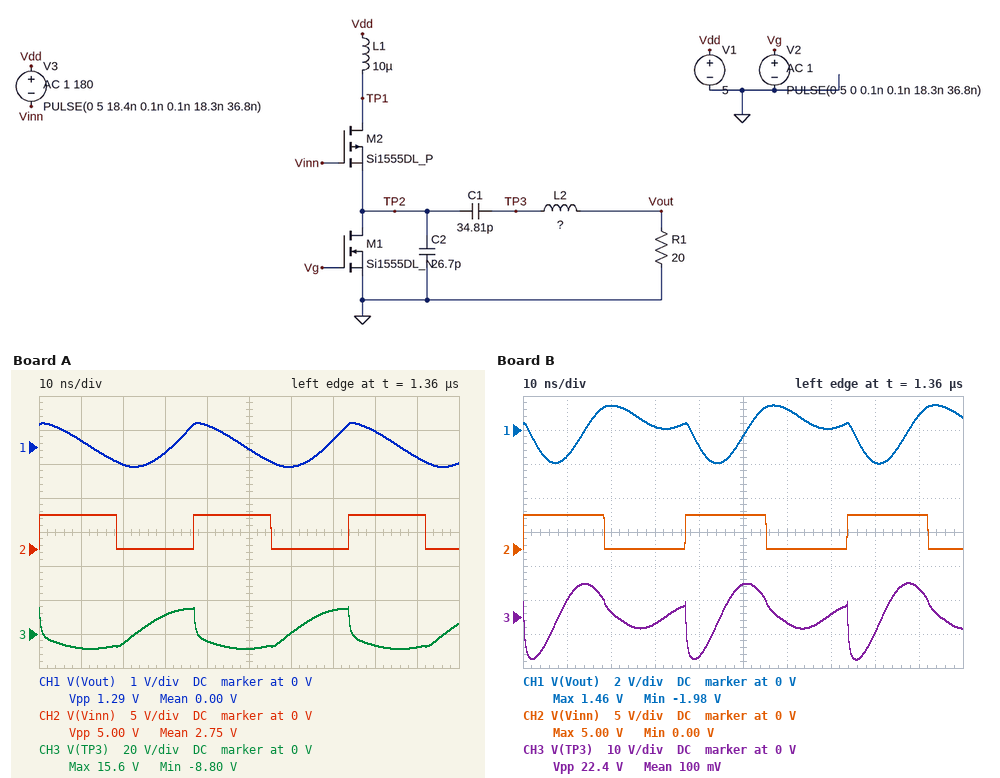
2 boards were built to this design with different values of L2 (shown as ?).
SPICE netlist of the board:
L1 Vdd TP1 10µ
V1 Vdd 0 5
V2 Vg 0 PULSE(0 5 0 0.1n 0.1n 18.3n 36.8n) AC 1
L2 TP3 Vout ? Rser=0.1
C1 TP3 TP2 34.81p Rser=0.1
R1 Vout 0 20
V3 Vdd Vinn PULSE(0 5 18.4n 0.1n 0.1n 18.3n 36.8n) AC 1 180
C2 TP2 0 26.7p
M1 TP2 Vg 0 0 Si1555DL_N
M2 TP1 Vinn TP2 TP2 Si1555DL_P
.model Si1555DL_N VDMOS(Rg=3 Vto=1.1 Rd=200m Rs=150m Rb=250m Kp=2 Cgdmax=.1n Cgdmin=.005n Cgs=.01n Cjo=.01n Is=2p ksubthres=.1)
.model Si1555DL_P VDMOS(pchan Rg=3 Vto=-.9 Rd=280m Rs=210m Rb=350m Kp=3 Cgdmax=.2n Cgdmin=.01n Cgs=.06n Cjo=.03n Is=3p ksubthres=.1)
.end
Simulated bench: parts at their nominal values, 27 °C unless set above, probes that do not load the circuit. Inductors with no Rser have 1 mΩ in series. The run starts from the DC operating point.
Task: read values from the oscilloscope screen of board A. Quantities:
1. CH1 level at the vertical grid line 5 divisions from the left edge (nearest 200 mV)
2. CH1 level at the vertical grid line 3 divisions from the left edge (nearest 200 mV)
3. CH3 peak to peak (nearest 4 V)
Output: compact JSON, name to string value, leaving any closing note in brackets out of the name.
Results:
{"CH1 level at the vertical grid line 5 divisions from the left edge": "0 V", "CH1 level at the vertical grid line 3 divisions from the left edge": "-200 mV", "CH3 peak to peak": "24 V"}
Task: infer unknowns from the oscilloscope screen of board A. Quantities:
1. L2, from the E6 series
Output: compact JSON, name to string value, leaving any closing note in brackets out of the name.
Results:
{"L2, from the E6 series": "2.2 µH"}
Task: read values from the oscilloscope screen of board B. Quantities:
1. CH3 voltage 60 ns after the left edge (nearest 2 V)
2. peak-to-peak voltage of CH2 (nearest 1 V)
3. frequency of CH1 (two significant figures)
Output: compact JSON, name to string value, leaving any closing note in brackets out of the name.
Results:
{"CH3 voltage 60 ns after the left edge": "-2 V", "peak-to-peak voltage of CH2": "5 V", "frequency of CH1": "27 MHz"}
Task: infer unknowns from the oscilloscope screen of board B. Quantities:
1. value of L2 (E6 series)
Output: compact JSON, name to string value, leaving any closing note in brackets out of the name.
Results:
{"value of L2": "470 nH"}
